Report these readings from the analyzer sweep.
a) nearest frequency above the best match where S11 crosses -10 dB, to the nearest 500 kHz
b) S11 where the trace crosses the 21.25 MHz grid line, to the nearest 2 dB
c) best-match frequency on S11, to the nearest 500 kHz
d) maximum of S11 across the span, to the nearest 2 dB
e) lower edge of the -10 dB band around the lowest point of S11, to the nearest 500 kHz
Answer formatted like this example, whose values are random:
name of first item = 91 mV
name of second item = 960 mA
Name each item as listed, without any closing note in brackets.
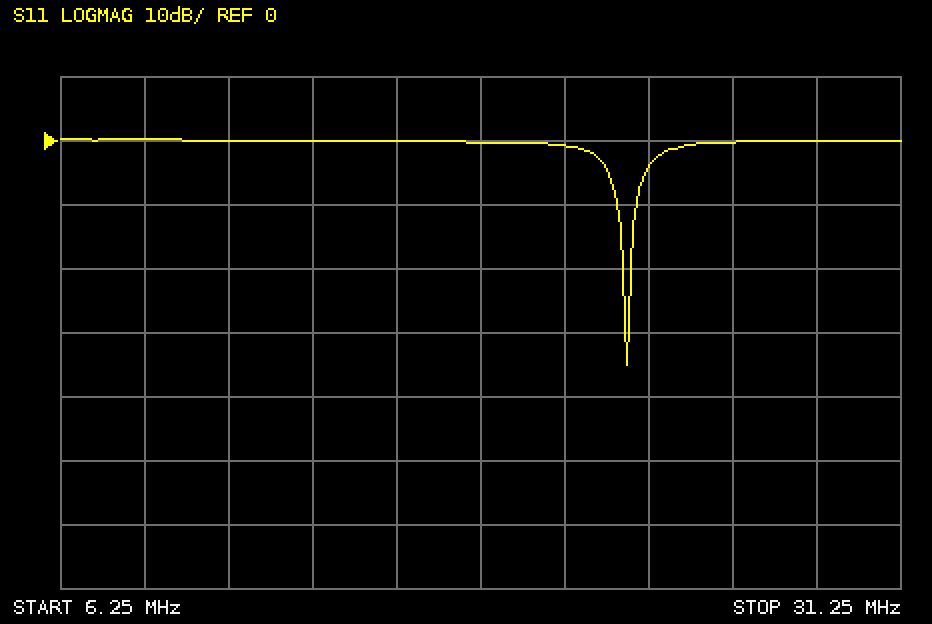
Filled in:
nearest frequency above the best match where S11 crosses -10 dB, to the nearest 500 kHz = 23.5 MHz
S11 where the trace crosses the 21.25 MHz grid line, to the nearest 2 dB = 0 dB
best-match frequency on S11, to the nearest 500 kHz = 23.0 MHz
maximum of S11 across the span, to the nearest 2 dB = 0 dB
lower edge of the -10 dB band around the lowest point of S11, to the nearest 500 kHz = 23.0 MHz
